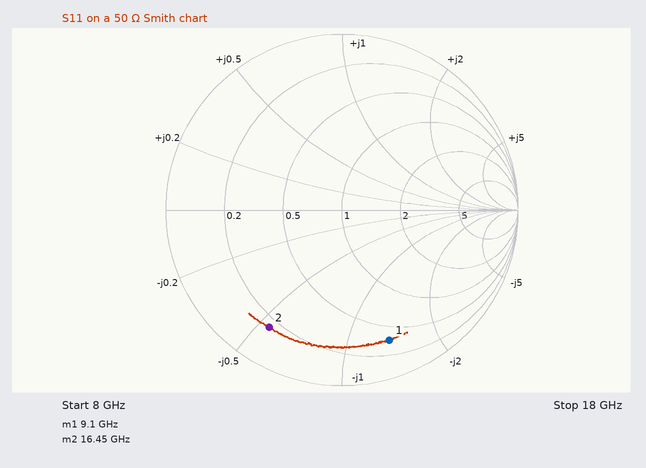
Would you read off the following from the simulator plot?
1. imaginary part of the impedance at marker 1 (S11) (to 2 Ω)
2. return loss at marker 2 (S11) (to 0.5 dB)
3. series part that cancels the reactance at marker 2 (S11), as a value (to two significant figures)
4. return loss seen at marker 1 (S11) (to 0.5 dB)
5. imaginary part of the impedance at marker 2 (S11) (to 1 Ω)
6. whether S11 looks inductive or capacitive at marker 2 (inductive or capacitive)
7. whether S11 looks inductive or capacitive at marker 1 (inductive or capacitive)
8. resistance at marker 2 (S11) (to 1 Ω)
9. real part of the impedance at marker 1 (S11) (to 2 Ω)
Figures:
-68 Ω
2.0 dB
260 pH
2.0 dB
-27 Ω
capacitive
capacitive
8 Ω
18 Ω
